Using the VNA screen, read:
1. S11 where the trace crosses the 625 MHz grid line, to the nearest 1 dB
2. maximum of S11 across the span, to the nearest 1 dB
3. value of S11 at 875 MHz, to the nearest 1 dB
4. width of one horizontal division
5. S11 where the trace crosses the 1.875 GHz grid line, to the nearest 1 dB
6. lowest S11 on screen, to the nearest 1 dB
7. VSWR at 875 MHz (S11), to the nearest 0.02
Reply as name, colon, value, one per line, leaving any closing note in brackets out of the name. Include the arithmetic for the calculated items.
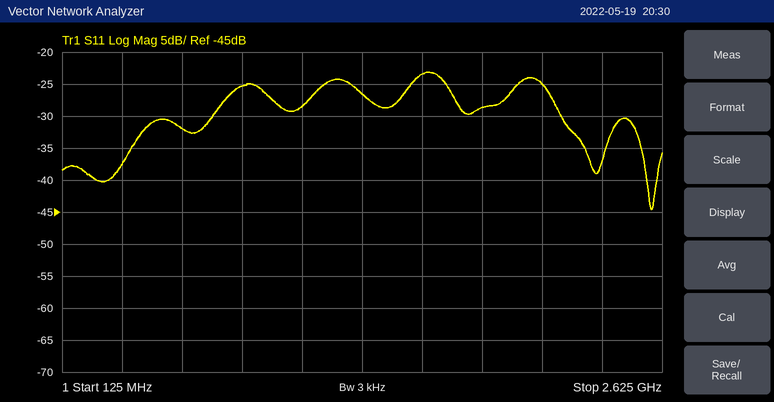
S11 where the trace crosses the 625 MHz grid line, to the nearest 1 dB: -32 dB
maximum of S11 across the span, to the nearest 1 dB: -23 dB
value of S11 at 875 MHz, to the nearest 1 dB: -25 dB
width of one horizontal division: 250 MHz
S11 where the trace crosses the 1.875 GHz grid line, to the nearest 1 dB: -29 dB
lowest S11 on screen, to the nearest 1 dB: -45 dB
VSWR at 875 MHz (S11), to the nearest 0.02: |Γ| = 10^(-25/20) = 0.0562; VSWR = (1 + 0.0562)/(1 − 0.0562) ≈ 1.12
